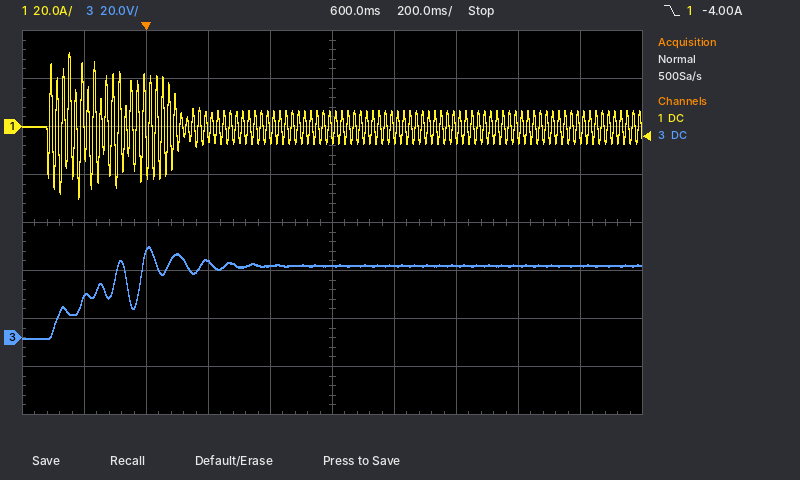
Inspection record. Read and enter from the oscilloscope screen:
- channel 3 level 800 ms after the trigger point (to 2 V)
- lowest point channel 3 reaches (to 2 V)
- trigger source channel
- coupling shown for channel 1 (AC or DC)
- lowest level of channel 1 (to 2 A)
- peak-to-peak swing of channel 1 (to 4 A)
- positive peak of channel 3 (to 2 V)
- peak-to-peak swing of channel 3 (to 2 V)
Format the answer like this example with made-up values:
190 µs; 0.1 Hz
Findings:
30 V; 0 V; channel 1; DC; -30 A; 60 A; 38 V; 38 V
